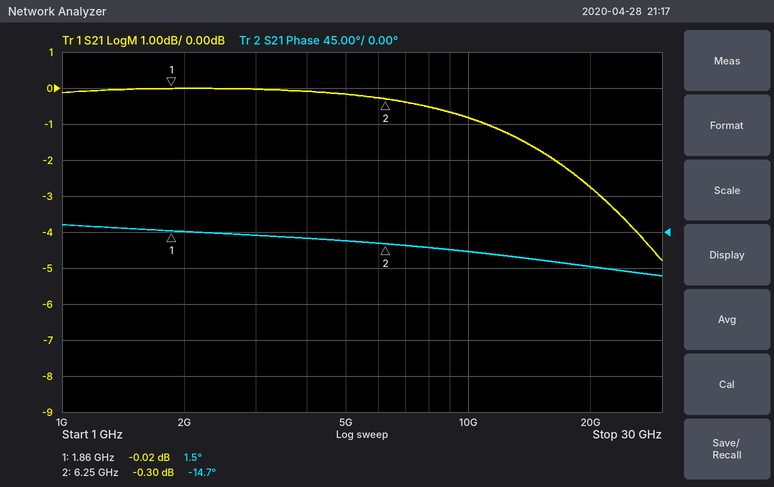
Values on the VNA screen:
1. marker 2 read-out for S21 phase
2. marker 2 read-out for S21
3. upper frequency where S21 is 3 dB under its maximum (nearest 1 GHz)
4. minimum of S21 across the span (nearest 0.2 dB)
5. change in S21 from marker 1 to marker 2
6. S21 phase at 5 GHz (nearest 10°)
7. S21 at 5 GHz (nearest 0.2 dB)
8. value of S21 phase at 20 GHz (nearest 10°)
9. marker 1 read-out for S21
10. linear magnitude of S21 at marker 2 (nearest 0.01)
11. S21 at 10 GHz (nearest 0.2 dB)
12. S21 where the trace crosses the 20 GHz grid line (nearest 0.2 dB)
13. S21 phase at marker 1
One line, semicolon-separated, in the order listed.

-14.7°; -0.30 dB; 21 GHz; -4.8 dB; -0.28 dB; -10°; -0.2 dB; -40°; -0.02 dB; 0.97; -0.8 dB; -2.8 dB; 1.5°
